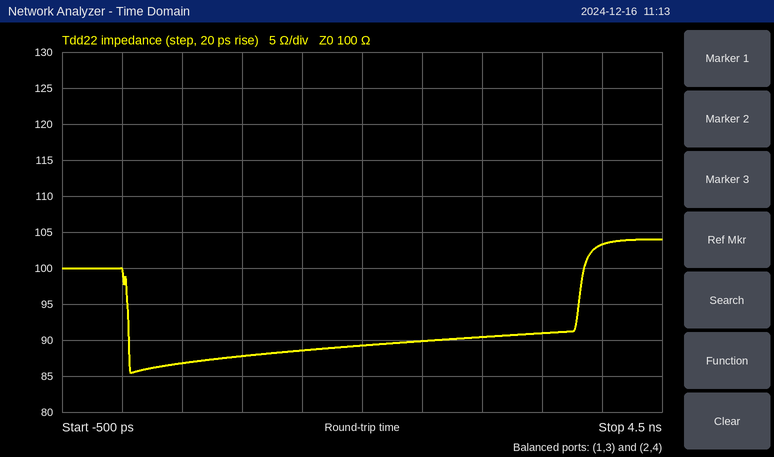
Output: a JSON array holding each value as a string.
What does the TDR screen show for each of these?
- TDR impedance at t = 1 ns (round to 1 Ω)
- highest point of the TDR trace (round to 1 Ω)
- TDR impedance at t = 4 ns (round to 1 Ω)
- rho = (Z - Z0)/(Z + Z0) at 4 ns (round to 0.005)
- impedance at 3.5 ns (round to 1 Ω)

["88 Ω", "104 Ω", "103 Ω", "+0.015", "91 Ω"]
